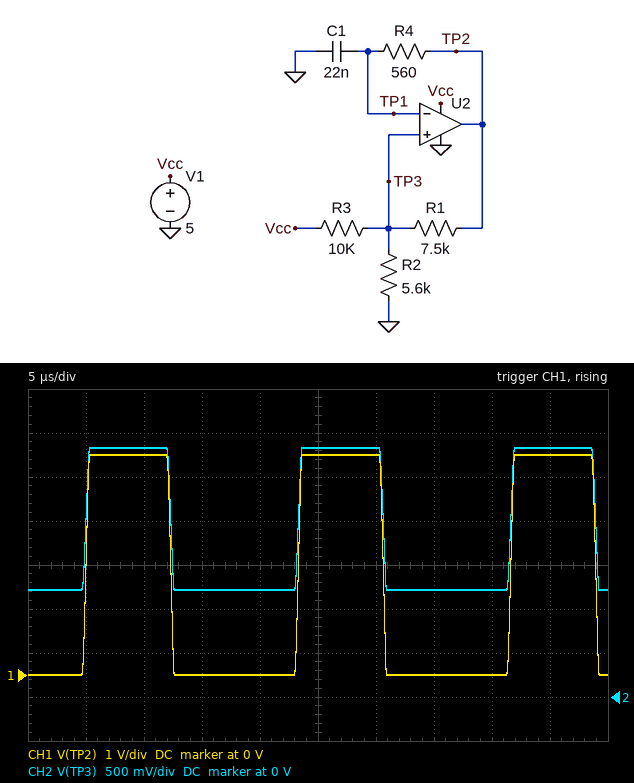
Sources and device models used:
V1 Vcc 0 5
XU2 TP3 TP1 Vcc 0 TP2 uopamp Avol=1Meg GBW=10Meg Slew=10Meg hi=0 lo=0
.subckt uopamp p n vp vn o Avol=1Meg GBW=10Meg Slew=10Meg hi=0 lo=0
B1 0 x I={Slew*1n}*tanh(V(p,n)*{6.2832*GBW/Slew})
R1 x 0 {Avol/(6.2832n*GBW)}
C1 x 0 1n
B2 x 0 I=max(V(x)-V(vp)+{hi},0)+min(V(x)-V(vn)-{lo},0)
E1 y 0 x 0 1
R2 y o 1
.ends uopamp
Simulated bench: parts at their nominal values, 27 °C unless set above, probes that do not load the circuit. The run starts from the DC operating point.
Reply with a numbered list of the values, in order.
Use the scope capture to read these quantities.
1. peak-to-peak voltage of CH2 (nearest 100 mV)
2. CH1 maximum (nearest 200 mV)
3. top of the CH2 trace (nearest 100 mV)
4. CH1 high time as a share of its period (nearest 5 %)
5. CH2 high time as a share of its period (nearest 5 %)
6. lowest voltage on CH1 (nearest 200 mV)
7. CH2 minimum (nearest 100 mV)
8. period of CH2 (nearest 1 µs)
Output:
1. 1.6 V
2. 5.0 V
3. 2.8 V
4. 40 %
5. 40 %
6. 0 V
7. 1.2 V
8. 18 µs
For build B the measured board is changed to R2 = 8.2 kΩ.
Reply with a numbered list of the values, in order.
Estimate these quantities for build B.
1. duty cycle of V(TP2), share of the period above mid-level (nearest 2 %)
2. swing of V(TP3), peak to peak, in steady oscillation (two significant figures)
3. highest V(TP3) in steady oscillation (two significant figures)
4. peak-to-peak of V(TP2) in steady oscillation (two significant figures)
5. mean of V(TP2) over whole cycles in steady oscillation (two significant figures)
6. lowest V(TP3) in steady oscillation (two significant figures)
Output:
1. 46 %
2. 1.9 V
3. 3.3 V
4. 5.0 V
5. 2.3 V
6. 1.4 V
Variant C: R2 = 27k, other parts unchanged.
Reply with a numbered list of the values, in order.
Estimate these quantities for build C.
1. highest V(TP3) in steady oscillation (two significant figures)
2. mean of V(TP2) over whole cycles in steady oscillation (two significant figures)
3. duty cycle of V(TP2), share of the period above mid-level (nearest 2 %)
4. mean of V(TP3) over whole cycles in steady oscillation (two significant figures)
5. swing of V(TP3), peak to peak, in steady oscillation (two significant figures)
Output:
1. 4.3 V
2. 3.2 V
3. 64 %
4. 3.4 V
5. 2.5 V
